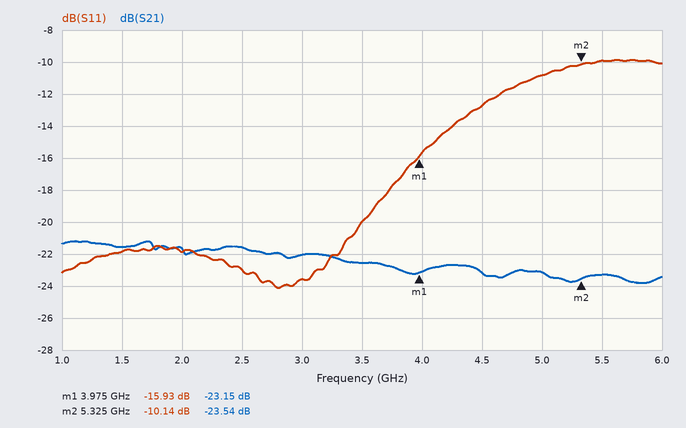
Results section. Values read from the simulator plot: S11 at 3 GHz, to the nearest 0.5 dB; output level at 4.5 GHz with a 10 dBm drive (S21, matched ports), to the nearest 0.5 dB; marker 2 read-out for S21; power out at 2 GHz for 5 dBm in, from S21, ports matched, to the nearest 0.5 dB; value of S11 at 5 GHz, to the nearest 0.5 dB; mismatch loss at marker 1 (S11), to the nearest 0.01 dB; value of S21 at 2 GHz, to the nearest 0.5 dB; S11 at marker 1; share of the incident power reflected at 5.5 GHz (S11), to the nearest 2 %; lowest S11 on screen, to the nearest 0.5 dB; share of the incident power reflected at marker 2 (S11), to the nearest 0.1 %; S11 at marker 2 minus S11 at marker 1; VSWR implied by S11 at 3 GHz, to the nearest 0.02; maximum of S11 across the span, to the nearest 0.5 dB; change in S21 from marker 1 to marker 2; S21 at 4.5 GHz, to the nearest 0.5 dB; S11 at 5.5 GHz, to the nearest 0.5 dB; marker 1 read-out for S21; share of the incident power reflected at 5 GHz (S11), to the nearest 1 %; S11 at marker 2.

-23.5 dB
-13.0 dBm
-23.54 dB
-16.5 dBm
-11.0 dB
0.11 dB
-21.5 dB
-15.93 dB
10 %
-24.0 dB
9.7 %
5.79 dB
1.14
-10.0 dB
-0.39 dB
-23.0 dB
-10.0 dB
-23.15 dB
8 %
-10.14 dB
